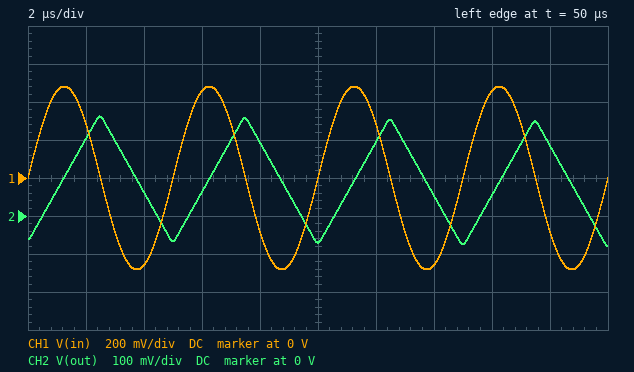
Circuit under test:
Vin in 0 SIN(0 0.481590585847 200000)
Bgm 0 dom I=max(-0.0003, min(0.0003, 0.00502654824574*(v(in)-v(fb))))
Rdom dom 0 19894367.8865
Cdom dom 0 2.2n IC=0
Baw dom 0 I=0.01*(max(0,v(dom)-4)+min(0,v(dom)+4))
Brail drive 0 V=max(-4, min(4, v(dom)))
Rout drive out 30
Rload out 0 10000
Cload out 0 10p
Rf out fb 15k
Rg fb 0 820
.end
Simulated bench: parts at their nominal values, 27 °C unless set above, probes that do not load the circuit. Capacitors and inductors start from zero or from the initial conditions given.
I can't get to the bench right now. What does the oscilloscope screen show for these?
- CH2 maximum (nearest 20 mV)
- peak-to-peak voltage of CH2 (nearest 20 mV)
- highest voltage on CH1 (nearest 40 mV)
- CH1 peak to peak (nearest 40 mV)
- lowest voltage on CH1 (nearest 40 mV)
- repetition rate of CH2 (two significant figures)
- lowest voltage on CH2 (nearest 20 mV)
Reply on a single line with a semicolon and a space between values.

260 mV; 340 mV; 480 mV; 960 mV; -480 mV; 200 kHz; -80 mV
